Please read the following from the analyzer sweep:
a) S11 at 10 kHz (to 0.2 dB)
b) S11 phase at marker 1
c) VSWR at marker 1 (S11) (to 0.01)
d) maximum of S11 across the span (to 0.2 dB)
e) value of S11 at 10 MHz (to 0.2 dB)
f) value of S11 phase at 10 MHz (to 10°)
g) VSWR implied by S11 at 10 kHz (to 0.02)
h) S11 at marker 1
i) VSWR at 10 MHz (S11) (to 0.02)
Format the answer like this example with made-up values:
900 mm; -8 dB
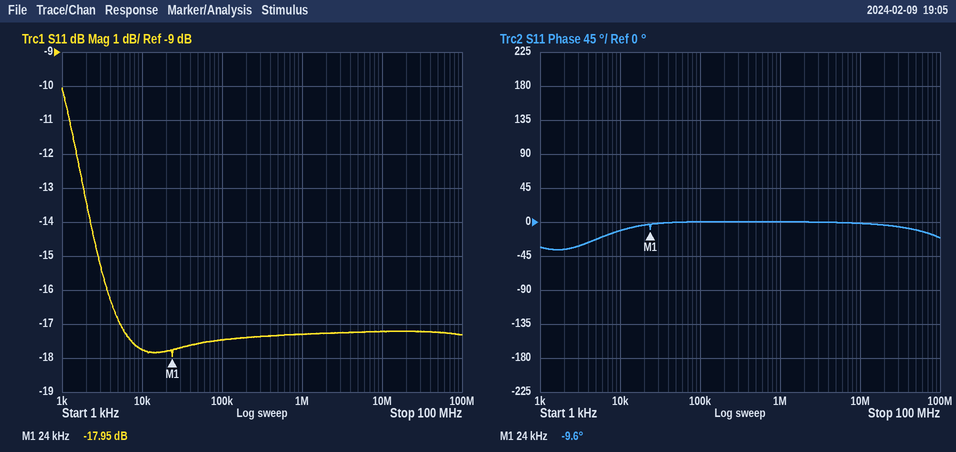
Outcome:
-17.8 dB; -9.6°; 1.29; -10.0 dB; -17.2 dB; 0°; 1.30; -17.95 dB; 1.32
